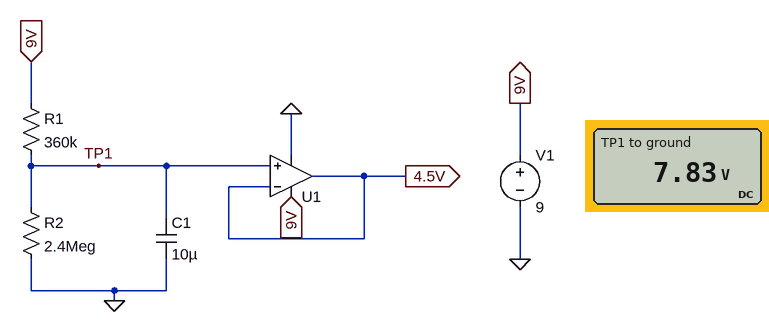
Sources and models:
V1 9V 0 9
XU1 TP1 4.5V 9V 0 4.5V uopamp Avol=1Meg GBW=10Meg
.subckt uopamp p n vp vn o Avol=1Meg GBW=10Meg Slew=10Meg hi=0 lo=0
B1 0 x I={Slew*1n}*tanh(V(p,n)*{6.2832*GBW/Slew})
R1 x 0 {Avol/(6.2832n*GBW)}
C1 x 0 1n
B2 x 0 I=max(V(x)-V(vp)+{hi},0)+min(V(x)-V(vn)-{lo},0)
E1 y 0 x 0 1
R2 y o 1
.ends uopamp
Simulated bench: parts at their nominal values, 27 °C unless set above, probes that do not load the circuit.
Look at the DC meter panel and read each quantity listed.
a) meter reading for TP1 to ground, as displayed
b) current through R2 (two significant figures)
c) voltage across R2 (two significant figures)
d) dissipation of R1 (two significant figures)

7.83 V
3.3 µA
7.8 V
3.8 µW
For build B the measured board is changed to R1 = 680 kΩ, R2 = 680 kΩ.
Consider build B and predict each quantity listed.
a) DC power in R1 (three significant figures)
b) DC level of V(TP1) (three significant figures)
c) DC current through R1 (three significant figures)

29.8 µW
4.50 V
6.62 µA
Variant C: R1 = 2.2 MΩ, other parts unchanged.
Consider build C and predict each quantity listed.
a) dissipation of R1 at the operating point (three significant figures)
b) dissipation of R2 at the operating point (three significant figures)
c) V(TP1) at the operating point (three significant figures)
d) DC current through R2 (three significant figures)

8.42 µW
9.19 µW
4.70 V
1.96 µA
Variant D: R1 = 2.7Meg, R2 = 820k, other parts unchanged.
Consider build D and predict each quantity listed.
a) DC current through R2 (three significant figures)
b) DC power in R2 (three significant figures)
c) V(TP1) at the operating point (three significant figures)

2.56 µA
5.36 µW
2.10 V
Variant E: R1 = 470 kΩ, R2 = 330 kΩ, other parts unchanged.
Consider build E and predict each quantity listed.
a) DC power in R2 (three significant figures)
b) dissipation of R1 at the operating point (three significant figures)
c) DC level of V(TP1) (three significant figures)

41.8 µW
59.5 µW
3.71 V
